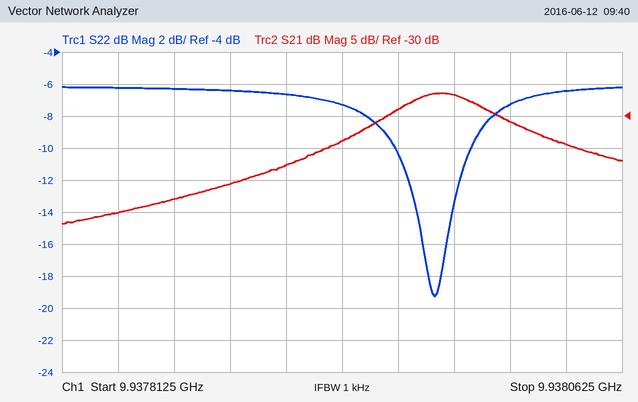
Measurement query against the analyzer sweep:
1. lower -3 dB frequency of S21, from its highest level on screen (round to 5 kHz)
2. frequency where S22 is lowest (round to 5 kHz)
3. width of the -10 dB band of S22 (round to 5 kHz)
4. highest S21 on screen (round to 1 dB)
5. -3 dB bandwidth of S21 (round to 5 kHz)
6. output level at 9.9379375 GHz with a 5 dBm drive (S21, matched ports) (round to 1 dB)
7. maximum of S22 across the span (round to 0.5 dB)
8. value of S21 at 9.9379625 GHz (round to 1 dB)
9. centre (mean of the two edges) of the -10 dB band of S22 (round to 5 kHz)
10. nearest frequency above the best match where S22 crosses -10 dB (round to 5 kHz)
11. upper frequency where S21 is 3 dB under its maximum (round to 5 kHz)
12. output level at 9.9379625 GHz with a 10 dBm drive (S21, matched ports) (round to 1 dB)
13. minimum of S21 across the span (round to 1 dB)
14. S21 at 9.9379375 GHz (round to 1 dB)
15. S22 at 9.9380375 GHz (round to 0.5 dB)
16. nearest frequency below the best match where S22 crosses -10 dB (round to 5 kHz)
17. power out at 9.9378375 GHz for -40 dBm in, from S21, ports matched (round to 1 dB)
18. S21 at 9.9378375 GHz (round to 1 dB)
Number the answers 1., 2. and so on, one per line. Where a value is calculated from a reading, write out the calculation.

1. 9.937960 GHz
2. 9.937980 GHz
3. 9.937995 GHz − 9.937960 GHz = 35 kHz
4. -26 dB
5. 9.938005 GHz − 9.937960 GHz = 45 kHz
6. 5 dBm + (-34 dB) = -29 dBm
7. -6.0 dB
8. -29 dB
9. 9.937980 GHz
10. 9.937995 GHz
11. 9.938005 GHz
12. 10 dBm + (-29 dB) = -19 dBm
13. -47 dB
14. -34 dB
15. -6.5 dB
16. 9.937960 GHz
17. -40 dBm + (-45 dB) = -85 dBm
18. -45 dB
